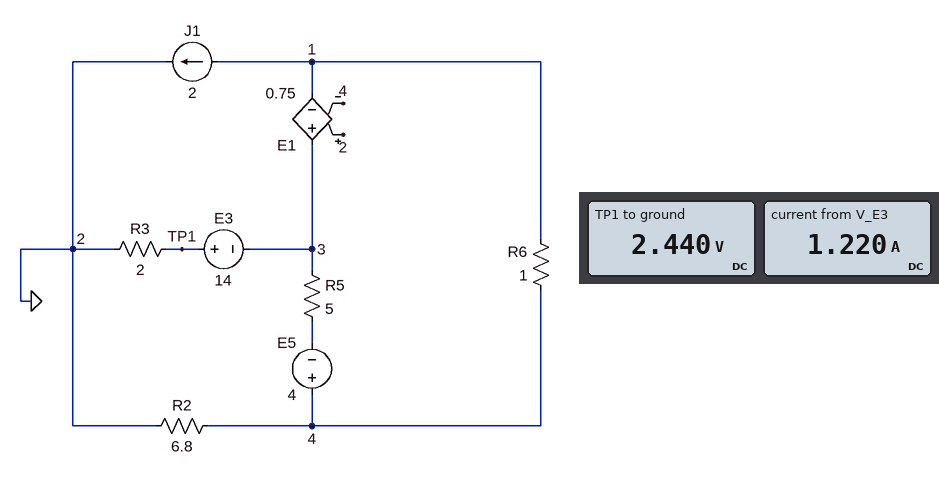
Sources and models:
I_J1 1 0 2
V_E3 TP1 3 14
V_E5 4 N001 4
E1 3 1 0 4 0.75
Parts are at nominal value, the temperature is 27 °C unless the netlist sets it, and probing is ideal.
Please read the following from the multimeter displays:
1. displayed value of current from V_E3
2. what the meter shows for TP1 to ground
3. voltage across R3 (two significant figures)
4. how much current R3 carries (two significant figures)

1.220 A
2.440 V
2.4 V
1.2 A
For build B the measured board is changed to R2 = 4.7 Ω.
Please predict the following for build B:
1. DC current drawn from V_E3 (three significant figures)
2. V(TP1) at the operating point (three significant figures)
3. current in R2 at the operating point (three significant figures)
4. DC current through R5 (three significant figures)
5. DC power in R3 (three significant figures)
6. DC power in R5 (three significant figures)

1.77 A
3.54 V
3.77 A
2.25 A
6.28 W
25.4 W
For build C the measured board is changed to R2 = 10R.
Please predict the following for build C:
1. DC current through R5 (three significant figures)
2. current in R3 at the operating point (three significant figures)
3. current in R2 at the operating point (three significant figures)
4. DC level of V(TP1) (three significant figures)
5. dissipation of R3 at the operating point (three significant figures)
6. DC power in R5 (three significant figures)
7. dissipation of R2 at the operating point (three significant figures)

3.52 A
633 mA
2.63 A
1.27 V
801 mW
61.9 W
69.3 W
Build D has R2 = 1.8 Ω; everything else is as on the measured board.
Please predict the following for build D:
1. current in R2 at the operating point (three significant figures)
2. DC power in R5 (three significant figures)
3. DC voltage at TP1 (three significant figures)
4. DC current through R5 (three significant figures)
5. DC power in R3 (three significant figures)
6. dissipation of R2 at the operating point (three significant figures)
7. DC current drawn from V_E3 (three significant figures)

4.94 A
4.56 W
5.88 V
955 mA
17.3 W
43.9 W
2.94 A
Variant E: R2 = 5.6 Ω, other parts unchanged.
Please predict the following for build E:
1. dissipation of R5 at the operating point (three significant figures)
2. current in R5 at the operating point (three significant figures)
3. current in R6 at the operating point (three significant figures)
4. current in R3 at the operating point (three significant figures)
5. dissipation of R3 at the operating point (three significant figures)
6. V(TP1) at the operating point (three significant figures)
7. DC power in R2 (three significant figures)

32.3 W
2.54 A
6.05 A
1.51 A
4.58 W
3.03 V
69.1 W
